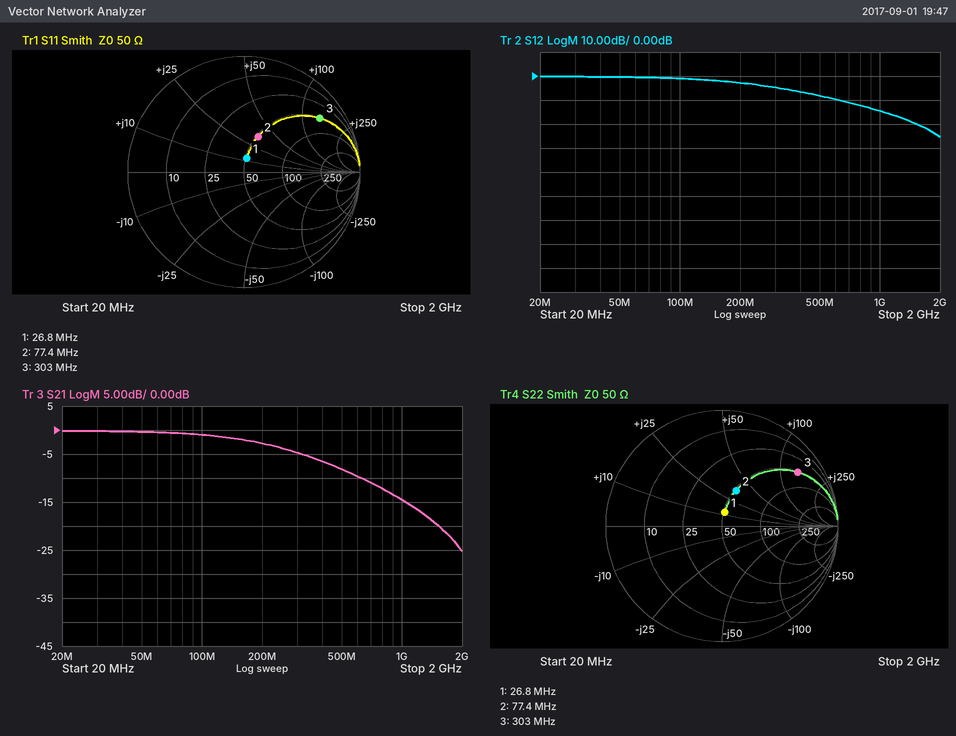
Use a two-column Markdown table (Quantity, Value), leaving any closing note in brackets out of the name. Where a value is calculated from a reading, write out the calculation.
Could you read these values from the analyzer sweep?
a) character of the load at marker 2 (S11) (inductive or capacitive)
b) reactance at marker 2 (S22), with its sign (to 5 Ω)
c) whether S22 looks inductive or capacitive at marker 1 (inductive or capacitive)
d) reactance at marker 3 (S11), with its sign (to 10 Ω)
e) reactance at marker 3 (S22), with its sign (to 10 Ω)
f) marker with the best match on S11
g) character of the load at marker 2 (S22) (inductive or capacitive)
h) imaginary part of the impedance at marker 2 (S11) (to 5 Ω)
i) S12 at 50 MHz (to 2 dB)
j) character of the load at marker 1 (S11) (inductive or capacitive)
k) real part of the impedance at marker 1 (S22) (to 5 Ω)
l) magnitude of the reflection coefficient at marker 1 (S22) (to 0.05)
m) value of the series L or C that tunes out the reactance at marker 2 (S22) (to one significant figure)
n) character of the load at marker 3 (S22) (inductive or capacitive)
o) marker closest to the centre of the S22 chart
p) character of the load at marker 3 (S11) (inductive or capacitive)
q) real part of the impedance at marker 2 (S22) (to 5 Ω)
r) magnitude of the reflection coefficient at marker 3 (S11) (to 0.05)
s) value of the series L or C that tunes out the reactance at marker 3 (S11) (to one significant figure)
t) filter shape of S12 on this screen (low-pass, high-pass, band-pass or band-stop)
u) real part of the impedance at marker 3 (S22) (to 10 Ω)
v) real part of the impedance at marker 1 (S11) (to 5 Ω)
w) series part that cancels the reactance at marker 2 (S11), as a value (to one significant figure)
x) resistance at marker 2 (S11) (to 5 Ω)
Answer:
| Quantity | Value |
|---|---|
| character of the load at marker 2 (S11) | inductive |
| reactance at marker 2 (S22), with its sign | +35 Ω |
| whether S22 looks inductive or capacitive at marker 1 | inductive |
| reactance at marker 3 (S11), with its sign | +140 Ω |
| reactance at marker 3 (S22), with its sign | +140 Ω |
| marker with the best match on S11 | marker 1 |
| character of the load at marker 2 (S22) | inductive |
| imaginary part of the impedance at marker 2 (S11) | +35 Ω |
| S12 at 50 MHz | 0 dB |
| character of the load at marker 1 (S11) | inductive |
| real part of the impedance at marker 1 (S22) | 50 Ω |
| magnitude of the reflection coefficient at marker 1 (S22) | 0.10 |
| value of the series L or C that tunes out the reactance at marker 2 (S22) | C = 1/(2π × 77.4 MHz × 35 Ω) ≈ 58.8 pF, so 60 pF to one significant figure |
| character of the load at marker 3 (S22) | inductive |
| marker closest to the centre of the S22 chart | marker 1 |
| character of the load at marker 3 (S11) | inductive |
| real part of the impedance at marker 2 (S22) | 50 Ω |
| magnitude of the reflection coefficient at marker 3 (S11) | 0.80 |
| value of the series L or C that tunes out the reactance at marker 3 (S11) | C = 1/(2π × 303 MHz × 140 Ω) ≈ 4 pF |
| filter shape of S12 on this screen | low-pass |
| real part of the impedance at marker 3 (S22) | 50 Ω |
| real part of the impedance at marker 1 (S11) | 50 Ω |
| series part that cancels the reactance at marker 2 (S11), as a value | C = 1/(2π × 77.4 MHz × 35 Ω) ≈ 58.8 pF, so 60 pF to one significant figure |
| resistance at marker 2 (S11) | 50 Ω |
